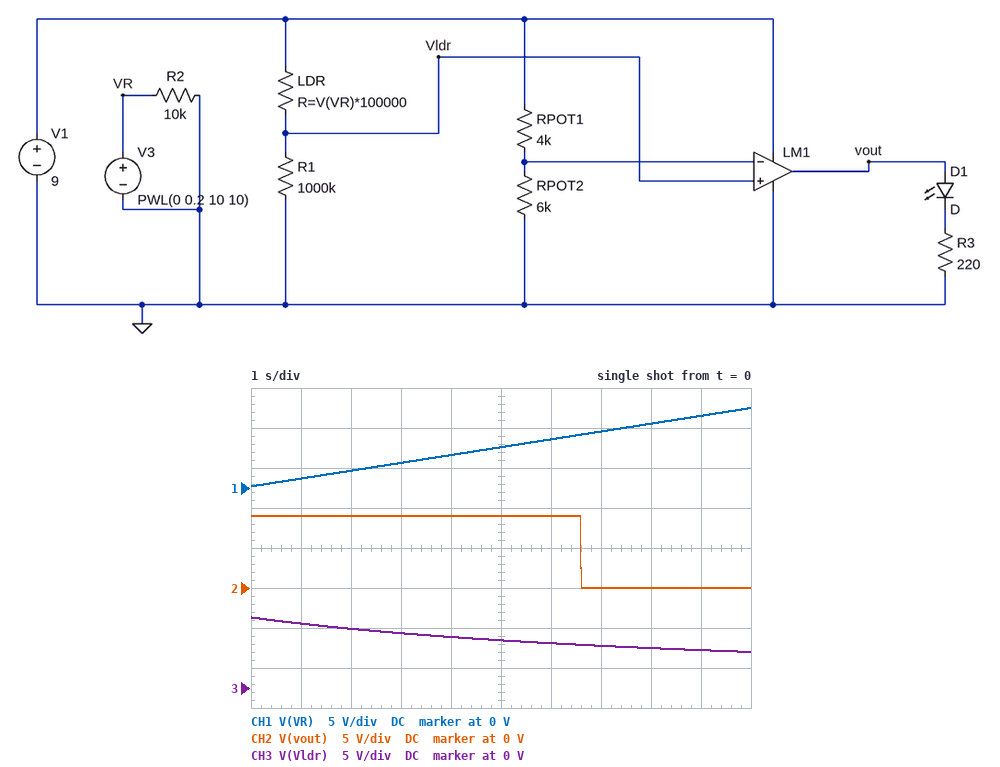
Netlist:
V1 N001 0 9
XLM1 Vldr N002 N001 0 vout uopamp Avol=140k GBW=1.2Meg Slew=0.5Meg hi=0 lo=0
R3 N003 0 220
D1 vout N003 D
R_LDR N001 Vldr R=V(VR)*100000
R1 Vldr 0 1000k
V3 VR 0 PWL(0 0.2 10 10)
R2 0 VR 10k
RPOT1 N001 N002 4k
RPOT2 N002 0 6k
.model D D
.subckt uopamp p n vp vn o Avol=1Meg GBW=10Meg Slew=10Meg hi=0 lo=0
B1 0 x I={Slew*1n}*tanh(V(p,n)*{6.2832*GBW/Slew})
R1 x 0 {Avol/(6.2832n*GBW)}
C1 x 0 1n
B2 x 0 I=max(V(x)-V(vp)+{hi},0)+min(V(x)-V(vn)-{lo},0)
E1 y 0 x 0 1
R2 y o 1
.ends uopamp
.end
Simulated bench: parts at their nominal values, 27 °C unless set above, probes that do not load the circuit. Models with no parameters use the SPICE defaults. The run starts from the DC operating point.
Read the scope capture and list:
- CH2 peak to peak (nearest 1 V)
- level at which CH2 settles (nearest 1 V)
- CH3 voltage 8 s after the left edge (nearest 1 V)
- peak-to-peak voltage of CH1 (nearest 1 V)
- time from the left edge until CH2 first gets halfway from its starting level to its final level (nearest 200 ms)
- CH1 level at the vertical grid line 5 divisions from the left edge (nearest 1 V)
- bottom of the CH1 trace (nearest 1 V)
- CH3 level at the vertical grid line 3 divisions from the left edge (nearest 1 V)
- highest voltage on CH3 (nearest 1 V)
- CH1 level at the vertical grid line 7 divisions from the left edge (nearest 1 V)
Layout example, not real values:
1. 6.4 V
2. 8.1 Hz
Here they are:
1. 9 V
2. 0 V
3. 5 V
4. 10 V
5. 6.6 s
6. 5 V
7. 0 V
8. 7 V
9. 9 V
10. 7 V
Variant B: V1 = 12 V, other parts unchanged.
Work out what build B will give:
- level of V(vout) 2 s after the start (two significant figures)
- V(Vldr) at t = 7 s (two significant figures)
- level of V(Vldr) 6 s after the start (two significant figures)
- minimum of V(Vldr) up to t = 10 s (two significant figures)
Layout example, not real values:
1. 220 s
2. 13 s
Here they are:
1. 12 V
2. 7.0 V
3. 7.5 V
4. 6.0 V
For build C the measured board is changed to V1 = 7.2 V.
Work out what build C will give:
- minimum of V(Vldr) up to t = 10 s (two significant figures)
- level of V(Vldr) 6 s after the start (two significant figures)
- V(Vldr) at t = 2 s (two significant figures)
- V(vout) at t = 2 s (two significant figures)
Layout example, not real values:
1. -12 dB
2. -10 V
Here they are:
1. 3.6 V
2. 4.5 V
3. 5.9 V
4. 7.2 V
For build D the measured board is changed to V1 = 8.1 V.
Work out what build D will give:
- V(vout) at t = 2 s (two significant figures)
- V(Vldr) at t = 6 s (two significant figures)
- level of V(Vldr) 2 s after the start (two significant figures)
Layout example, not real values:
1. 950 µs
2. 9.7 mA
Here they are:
1. 8.1 V
2. 5.0 V
3. 6.7 V
